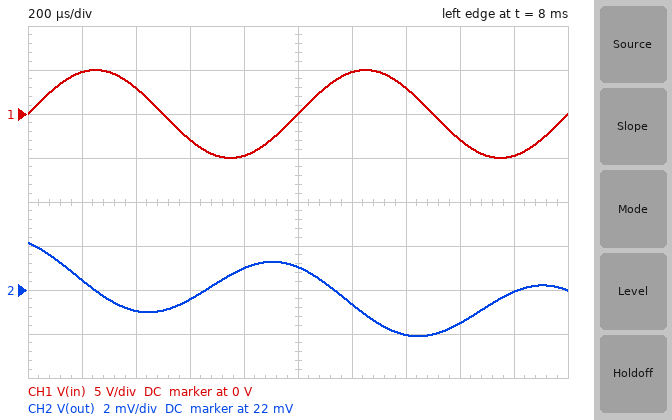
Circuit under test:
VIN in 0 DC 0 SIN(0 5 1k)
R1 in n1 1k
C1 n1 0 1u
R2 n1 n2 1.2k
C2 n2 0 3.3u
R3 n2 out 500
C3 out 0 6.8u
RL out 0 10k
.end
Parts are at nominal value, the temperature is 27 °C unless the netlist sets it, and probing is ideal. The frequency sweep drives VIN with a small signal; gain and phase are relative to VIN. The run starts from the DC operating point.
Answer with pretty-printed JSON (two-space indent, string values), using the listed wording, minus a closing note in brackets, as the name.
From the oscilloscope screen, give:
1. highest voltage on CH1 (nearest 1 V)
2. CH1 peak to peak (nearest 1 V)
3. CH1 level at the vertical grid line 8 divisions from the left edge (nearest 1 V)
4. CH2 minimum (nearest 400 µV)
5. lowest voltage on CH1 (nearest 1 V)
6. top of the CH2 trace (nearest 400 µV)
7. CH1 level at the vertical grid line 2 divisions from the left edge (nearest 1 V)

{
  "highest voltage on CH1": "5 V",
  "CH1 peak to peak": "10 V",
  "CH1 level at the vertical grid line 8 divisions from the left edge": "-3 V",
  "CH2 minimum": "20.0 mV",
  "lowest voltage on CH1": "-5 V",
  "top of the CH2 trace": "24.0 mV",
  "CH1 level at the vertical grid line 2 divisions from the left edge": "3 V"
}
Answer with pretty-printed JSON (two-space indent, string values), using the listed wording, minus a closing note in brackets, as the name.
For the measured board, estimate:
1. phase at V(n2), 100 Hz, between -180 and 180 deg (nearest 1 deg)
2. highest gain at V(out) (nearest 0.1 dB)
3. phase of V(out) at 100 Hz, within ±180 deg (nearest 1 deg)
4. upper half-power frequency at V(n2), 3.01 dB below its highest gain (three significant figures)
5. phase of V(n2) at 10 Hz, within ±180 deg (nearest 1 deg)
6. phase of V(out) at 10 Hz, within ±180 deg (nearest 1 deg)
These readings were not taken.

{
  "phase at V(n2), 100 Hz, between -180 and 180 deg": "-73 deg",
  "highest gain at V(out)": "-2.1 dB",
  "phase of V(out) at 100 Hz, within ±180 deg": "-137 deg",
  "upper half-power frequency at V(n2), 3.01 dB below its highest gain": "8.23 Hz",
  "phase of V(n2) at 10 Hz, within ±180 deg": "-45 deg",
  "phase of V(out) at 10 Hz, within ±180 deg": "-57 deg"
}
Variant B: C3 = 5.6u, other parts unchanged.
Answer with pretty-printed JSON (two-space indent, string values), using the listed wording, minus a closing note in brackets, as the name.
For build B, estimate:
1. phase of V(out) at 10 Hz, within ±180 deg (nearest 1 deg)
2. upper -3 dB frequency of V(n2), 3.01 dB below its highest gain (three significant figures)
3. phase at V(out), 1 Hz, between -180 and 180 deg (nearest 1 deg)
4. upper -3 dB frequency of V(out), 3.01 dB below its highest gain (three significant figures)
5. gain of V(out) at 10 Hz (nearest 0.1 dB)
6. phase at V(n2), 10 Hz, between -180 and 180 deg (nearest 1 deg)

{
  "phase of V(out) at 10 Hz, within ±180 deg": "-53 deg",
  "upper -3 dB frequency of V(n2), 3.01 dB below its highest gain": "9.38 Hz",
  "phase at V(out), 1 Hz, between -180 and 180 deg": "-7 deg",
  "upper -3 dB frequency of V(out), 3.01 dB below its highest gain": "9.15 Hz",
  "gain of V(out) at 10 Hz": "-5.5 dB",
  "phase at V(n2), 10 Hz, between -180 and 180 deg": "-43 deg"
}
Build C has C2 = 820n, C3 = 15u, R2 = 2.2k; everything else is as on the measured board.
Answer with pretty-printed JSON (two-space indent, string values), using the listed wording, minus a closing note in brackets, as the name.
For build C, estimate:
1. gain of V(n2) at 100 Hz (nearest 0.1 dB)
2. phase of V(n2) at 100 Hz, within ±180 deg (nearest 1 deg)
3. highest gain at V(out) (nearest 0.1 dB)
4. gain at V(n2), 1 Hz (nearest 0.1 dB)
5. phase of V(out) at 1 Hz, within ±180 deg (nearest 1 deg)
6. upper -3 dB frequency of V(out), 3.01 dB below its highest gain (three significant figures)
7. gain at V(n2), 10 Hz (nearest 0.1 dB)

{
  "gain of V(n2) at 100 Hz": "-18.6 dB",
  "phase of V(n2) at 100 Hz, within ±180 deg": "-47 deg",
  "highest gain at V(out)": "-2.7 dB",
  "gain at V(n2), 1 Hz": "-2.6 dB",
  "phase of V(out) at 1 Hz, within ±180 deg": "-15 deg",
  "upper -3 dB frequency of V(out), 3.01 dB below its highest gain": "3.75 Hz",
  "gain at V(n2), 10 Hz": "-10.6 dB"
}
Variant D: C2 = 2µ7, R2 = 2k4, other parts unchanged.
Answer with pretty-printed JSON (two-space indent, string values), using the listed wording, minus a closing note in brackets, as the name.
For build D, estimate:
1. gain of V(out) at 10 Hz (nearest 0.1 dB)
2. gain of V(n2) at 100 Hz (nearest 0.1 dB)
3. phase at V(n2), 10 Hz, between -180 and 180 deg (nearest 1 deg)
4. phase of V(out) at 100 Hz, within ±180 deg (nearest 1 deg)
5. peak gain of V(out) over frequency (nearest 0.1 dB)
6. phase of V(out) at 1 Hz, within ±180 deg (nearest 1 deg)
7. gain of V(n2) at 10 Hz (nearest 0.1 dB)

{
  "gain of V(out) at 10 Hz": "-8.4 dB",
  "gain of V(n2) at 100 Hz": "-21.4 dB",
  "phase at V(n2), 10 Hz, between -180 and 180 deg": "-52 deg",
  "phase of V(out) at 100 Hz, within ±180 deg": "-140 deg",
  "peak gain of V(out) over frequency": "-2.9 dB",
  "phase of V(out) at 1 Hz, within ±180 deg": "-10 deg",
  "gain of V(n2) at 10 Hz": "-7.8 dB"
}
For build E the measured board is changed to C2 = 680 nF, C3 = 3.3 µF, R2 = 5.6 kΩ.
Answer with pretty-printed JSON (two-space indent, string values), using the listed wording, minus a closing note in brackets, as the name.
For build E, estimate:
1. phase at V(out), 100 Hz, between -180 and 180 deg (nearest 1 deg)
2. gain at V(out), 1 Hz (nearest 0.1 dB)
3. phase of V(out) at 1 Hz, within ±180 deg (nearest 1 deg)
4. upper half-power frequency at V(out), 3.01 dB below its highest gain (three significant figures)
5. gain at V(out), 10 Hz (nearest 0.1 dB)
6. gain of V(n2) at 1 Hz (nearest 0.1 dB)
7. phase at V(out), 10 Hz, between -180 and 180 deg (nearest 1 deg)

{
  "phase at V(out), 100 Hz, between -180 and 180 deg": "-122 deg",
  "gain at V(out), 1 Hz": "-4.7 dB",
  "phase of V(out) at 1 Hz, within ±180 deg": "-6 deg",
  "upper half-power frequency at V(out), 3.01 dB below its highest gain": "9.75 Hz",
  "gain at V(out), 10 Hz": "-7.8 dB",
  "gain of V(n2) at 1 Hz": "-4.3 dB",
  "phase at V(out), 10 Hz, between -180 and 180 deg": "-50 deg"
}
